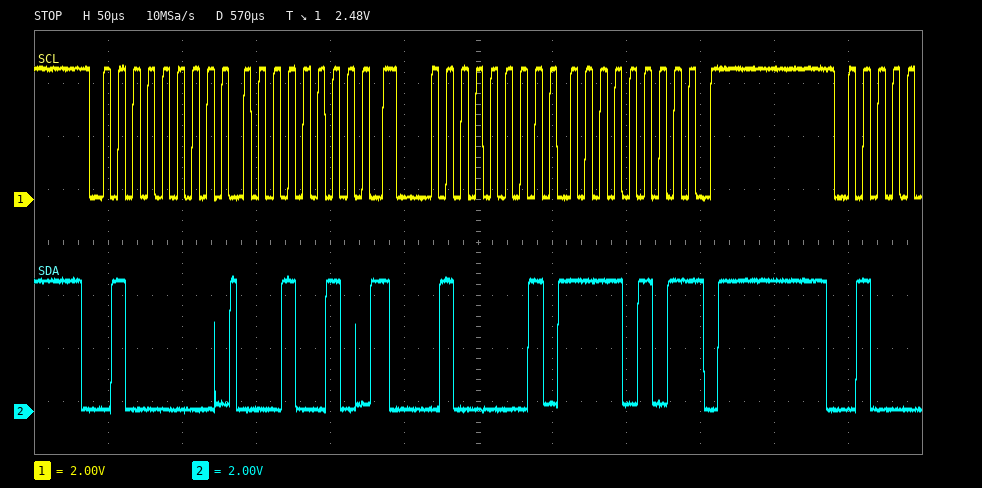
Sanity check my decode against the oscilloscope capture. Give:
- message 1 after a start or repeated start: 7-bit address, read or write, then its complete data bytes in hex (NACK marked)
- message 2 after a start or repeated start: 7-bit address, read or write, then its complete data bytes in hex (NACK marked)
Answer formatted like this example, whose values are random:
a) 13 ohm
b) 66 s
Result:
a) 0x20 write: 12
b) 0x20 read: F5 NACK
